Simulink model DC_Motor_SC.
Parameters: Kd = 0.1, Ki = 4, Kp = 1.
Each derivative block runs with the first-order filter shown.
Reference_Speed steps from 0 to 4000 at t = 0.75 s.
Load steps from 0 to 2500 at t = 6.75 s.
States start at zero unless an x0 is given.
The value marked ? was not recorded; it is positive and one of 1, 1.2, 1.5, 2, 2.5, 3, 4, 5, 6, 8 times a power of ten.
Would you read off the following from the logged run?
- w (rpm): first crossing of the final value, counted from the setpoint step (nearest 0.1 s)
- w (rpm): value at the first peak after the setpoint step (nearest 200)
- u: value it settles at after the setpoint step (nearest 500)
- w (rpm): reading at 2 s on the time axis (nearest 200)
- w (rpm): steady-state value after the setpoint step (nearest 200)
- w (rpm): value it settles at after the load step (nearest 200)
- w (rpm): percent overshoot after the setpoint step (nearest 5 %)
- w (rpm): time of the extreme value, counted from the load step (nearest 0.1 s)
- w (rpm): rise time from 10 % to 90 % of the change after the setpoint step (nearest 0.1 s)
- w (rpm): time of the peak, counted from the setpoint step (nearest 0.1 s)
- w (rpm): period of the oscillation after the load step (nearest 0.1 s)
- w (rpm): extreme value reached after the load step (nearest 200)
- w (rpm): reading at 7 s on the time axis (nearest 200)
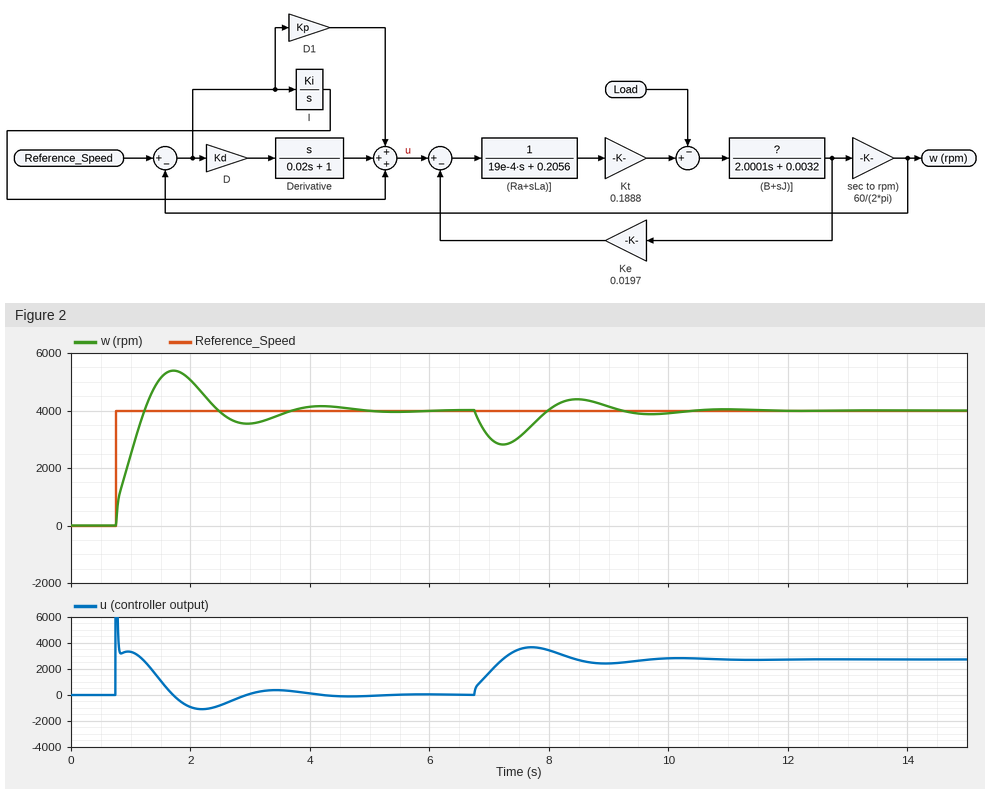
0.5 s
5400
0
5000
4000
4000
35 %
0.5 s
0.4 s
1.0 s
2.5 s
2800
3000
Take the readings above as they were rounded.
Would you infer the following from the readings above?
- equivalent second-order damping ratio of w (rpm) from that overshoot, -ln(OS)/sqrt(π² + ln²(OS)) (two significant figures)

0.32
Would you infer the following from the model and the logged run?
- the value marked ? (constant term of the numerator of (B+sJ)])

0.5
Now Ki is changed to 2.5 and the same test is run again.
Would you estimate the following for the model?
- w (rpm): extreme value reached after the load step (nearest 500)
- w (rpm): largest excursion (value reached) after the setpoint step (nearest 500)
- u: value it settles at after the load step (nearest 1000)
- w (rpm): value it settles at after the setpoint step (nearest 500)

2500
5000
3000
4000
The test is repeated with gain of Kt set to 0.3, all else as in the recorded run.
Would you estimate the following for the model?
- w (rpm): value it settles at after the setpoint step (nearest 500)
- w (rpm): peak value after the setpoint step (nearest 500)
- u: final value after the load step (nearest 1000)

4000
5000
2000
